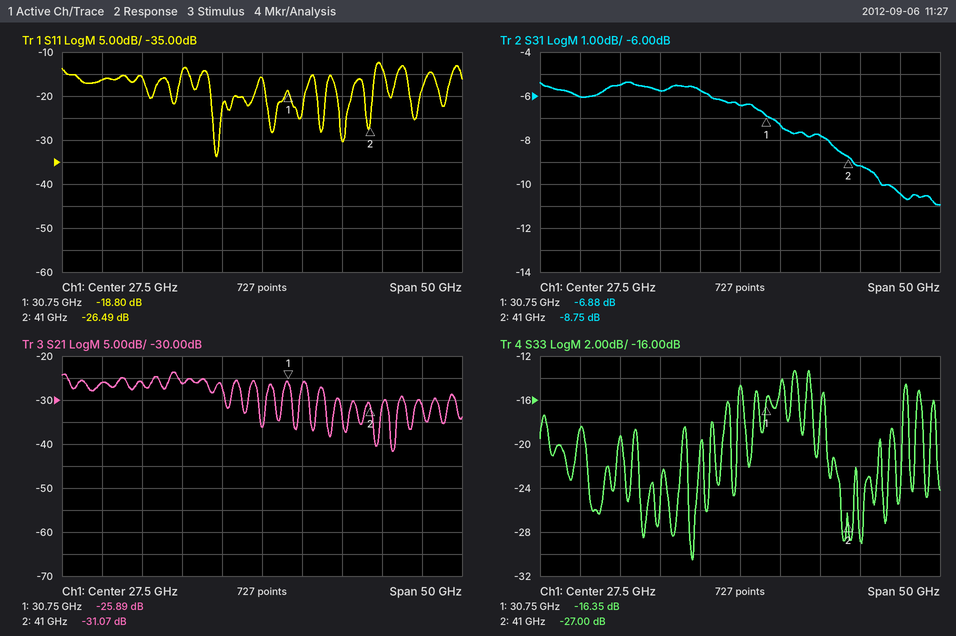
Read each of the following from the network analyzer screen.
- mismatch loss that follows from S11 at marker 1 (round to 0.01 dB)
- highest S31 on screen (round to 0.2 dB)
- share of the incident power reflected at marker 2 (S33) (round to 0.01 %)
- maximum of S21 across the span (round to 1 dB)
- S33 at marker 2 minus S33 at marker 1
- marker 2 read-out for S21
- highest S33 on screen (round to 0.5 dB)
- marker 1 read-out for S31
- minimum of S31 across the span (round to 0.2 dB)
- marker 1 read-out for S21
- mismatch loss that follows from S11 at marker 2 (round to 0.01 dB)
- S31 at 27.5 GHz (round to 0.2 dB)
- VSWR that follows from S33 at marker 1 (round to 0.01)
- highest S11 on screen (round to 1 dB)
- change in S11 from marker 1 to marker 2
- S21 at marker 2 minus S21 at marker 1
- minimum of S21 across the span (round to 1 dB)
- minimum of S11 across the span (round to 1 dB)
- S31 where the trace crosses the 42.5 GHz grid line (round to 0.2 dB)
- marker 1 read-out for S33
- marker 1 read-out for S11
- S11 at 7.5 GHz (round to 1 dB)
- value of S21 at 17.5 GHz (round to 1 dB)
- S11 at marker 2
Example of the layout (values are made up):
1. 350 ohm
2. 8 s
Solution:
1. 0.06 dB
2. -5.4 dB
3. 0.20 %
4. -24 dB
5. -10.65 dB
6. -31.07 dB
7. -13.5 dB
8. -6.88 dB
9. -11.0 dB
10. -25.89 dB
11. 0.01 dB
12. -6.4 dB
13. 1.36
14. -12 dB
15. -7.69 dB
16. -5.18 dB
17. -42 dB
18. -34 dB
19. -9.2 dB
20. -16.35 dB
21. -18.80 dB
22. -16 dB
23. -26 dB
24. -26.49 dB
